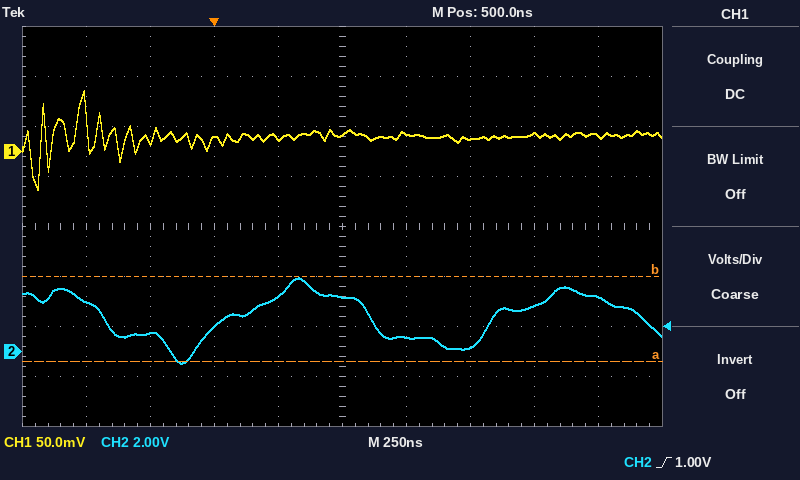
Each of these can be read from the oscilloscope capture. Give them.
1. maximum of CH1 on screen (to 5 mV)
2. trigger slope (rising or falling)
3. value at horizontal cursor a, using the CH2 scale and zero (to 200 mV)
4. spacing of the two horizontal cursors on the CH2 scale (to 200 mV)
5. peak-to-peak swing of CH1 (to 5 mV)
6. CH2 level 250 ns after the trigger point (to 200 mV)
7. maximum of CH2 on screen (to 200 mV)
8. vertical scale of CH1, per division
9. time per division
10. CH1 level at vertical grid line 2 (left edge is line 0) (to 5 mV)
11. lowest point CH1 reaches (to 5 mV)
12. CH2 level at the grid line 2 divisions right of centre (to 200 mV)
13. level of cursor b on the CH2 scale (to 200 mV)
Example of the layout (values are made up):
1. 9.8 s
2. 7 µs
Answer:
1. 60 mV
2. rising
3. -400 mV
4. 3.4 V
5. 100 mV
6. 2.2 V
7. 3.0 V
8. 50 mV
9. 250 ns
10. 10 mV
11. -40 mV
12. 200 mV
13. 3.0 V
